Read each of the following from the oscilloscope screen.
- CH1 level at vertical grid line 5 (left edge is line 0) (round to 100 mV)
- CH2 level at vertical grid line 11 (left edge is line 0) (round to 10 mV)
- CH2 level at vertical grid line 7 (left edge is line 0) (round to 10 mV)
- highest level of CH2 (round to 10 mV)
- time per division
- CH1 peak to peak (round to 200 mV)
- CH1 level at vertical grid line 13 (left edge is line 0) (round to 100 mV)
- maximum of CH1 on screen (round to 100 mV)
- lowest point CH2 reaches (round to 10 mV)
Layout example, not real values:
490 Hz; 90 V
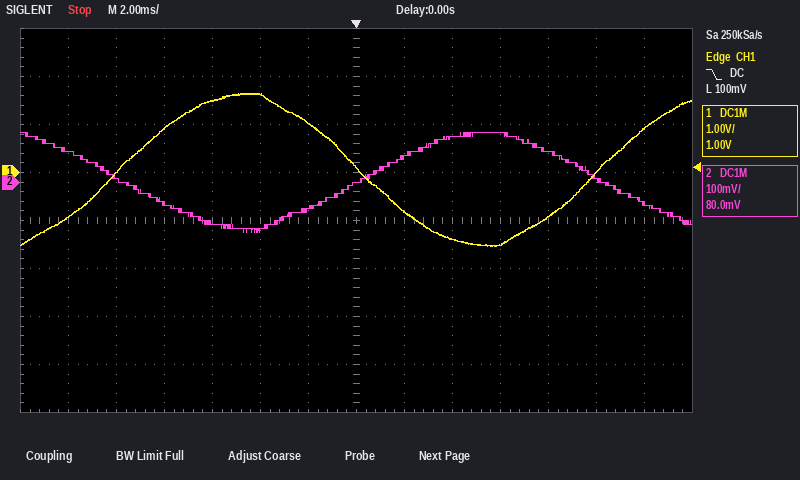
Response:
1.6 V; 60 mV; 0 mV; 100 mV; 2 ms; 3.2 V; 900 mV; 1.6 V; -100 mV
